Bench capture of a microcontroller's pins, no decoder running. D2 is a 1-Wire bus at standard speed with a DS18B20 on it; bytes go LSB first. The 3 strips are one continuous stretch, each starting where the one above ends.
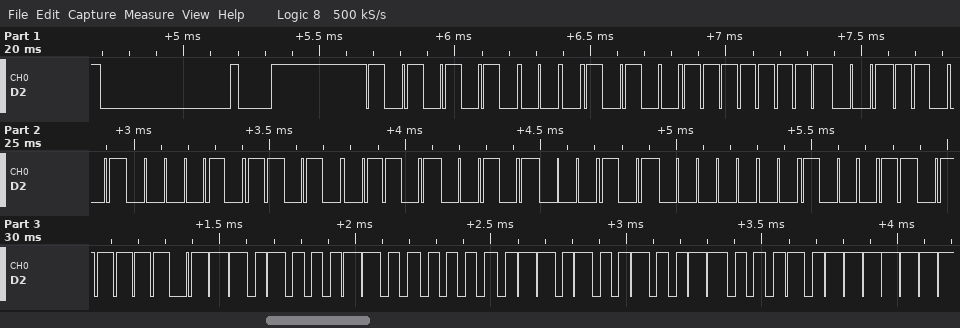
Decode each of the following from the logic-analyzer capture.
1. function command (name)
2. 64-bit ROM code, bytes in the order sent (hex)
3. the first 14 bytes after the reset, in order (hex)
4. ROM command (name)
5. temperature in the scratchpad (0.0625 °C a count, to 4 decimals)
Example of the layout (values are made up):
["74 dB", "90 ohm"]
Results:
["Read Scratchpad", "28 FF 9C D0 B2 14 05 C4", "55 28 FF 9C D0 B2 14 05 C4 BE 8B 01 4B 46", "Match ROM", "24.6875 °C"]
